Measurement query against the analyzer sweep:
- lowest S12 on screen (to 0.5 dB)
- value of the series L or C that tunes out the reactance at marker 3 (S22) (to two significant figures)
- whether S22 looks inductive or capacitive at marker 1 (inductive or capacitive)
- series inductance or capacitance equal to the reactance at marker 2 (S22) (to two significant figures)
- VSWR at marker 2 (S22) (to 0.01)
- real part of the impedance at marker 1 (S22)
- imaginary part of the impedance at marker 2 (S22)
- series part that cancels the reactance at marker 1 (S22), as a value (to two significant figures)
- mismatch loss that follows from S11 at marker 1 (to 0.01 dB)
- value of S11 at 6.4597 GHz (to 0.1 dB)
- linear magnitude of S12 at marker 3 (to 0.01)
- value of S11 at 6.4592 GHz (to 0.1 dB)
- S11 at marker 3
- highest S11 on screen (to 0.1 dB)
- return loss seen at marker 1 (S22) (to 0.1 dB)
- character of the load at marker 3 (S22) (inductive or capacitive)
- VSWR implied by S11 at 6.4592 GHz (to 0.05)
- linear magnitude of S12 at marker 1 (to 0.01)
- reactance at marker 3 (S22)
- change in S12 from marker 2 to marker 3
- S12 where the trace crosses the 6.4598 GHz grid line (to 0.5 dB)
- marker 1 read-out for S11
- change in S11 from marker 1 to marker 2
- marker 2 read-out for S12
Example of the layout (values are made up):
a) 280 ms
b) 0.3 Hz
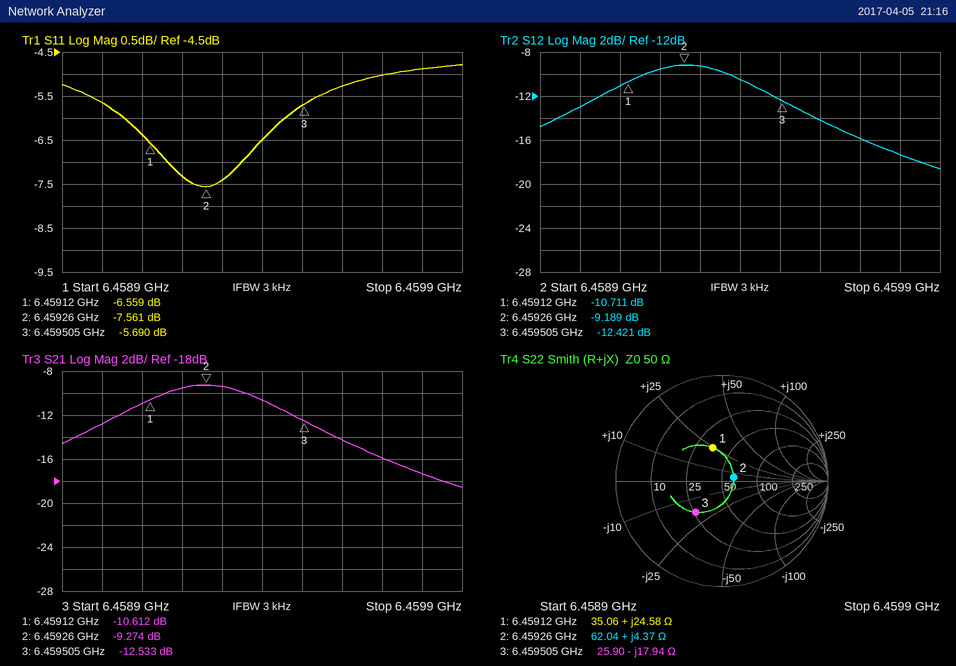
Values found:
a) -18.5 dB
b) 440 pH
c) inductive
d) 110 pH
e) 1.26
f) 35.06 Ω
g) +4.37 Ω
h) 1.0 pF
i) 1.08 dB
j) -5.0 dB
k) 0.24
l) -7.3 dB
m) -5.690 dB
n) -4.8 dB
o) 9.8 dB
p) capacitive
q) 2.50
r) 0.29
s) -17.94 Ω
t) -3.232 dB
u) -17.5 dB
v) -6.559 dB
w) -1.002 dB
x) -9.189 dB
